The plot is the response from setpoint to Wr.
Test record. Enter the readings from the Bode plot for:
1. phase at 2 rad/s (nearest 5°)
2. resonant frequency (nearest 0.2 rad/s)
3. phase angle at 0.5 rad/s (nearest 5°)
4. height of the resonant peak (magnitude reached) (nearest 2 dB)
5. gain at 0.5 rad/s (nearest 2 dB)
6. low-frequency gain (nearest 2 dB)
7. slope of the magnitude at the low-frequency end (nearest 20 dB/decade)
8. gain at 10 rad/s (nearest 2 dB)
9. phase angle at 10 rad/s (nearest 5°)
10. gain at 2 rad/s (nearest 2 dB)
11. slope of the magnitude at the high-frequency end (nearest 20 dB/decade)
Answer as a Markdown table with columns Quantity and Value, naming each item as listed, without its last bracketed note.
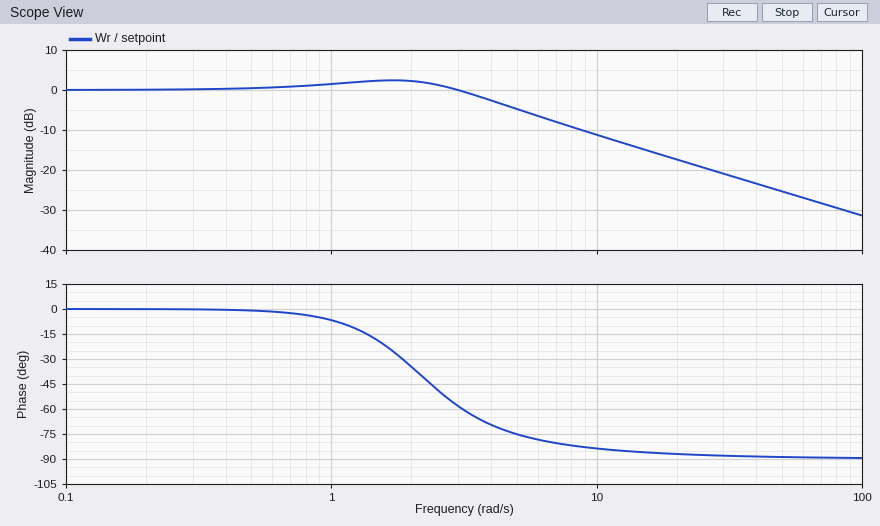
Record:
| Quantity | Value |
|---|---|
| phase at 2 rad/s | -35° |
| resonant frequency | 1.6 rad/s |
| phase angle at 0.5 rad/s | 0° |
| height of the resonant peak (magnitude reached) | 2 dB |
| gain at 0.5 rad/s | 0 dB |
| low-frequency gain | 0 dB |
| slope of the magnitude at the low-frequency end | 0 dB/decade |
| gain at 10 rad/s | -12 dB |
| phase angle at 10 rad/s | -85° |
| gain at 2 rad/s | 2 dB |
| slope of the magnitude at the high-frequency end | -20 dB/decade |
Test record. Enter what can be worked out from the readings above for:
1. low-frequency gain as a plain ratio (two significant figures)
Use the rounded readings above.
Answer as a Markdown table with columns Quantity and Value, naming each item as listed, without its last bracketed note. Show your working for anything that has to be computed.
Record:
| Quantity | Value |
|---|---|
| low-frequency gain as a plain ratio | 10^(0 / 20) = 1.0 |
